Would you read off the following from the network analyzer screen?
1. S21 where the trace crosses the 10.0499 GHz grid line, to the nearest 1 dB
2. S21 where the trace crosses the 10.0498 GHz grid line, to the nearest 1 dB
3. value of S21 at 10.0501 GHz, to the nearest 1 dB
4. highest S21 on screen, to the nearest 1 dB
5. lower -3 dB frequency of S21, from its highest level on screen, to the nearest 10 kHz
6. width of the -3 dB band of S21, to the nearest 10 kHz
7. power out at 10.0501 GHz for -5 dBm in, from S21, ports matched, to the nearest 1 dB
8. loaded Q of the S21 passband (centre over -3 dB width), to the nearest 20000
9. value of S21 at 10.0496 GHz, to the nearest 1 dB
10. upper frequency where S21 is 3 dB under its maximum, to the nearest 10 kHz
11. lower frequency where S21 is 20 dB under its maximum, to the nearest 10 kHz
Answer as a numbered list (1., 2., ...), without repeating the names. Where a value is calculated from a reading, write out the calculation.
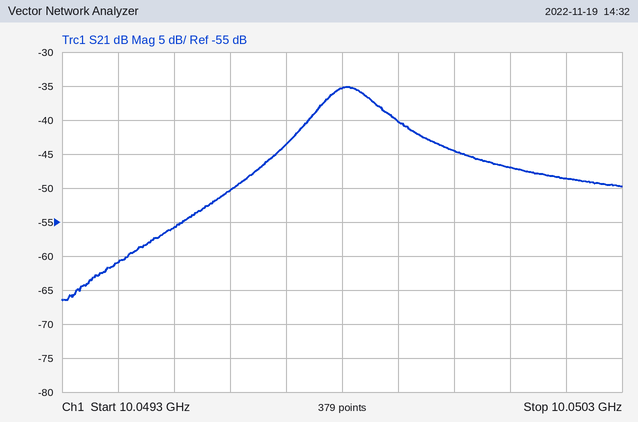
1. -40 dB
2. -35 dB
3. -47 dB
4. -35 dB
5. 10.04976 GHz
6. 10.04987 GHz − 10.04976 GHz = 110 kHz
7. -5 dBm + (-47 dB) = -52 dBm
8. 10.0498 GHz / 110 kHz ≈ 91362, so 100000 to the nearest 20000
9. -50 dB
10. 10.04987 GHz
11. 10.04951 GHz
